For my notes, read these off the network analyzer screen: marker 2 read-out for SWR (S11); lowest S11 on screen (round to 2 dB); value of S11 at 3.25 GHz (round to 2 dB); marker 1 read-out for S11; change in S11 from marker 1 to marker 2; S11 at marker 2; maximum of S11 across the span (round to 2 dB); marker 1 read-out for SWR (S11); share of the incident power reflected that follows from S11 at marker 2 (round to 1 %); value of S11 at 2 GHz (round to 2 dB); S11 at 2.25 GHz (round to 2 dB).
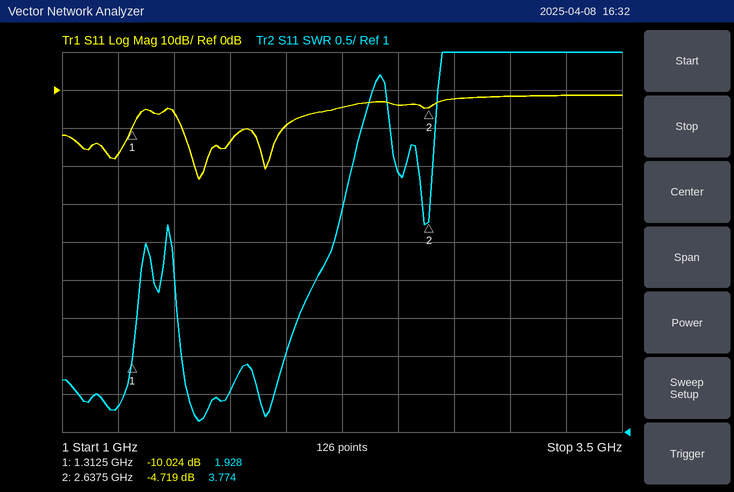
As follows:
3.774
-24 dB
-2 dB
-10.024 dB
5.305 dB
-4.719 dB
-2 dB
1.928
34 %
-10 dB
-4 dB
